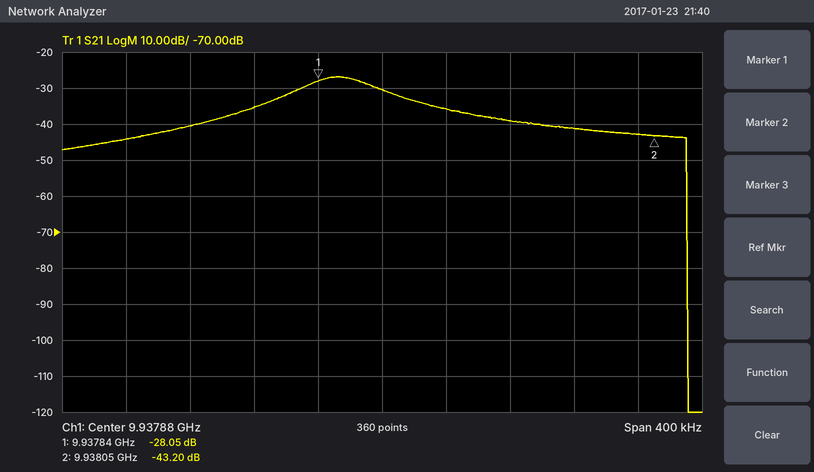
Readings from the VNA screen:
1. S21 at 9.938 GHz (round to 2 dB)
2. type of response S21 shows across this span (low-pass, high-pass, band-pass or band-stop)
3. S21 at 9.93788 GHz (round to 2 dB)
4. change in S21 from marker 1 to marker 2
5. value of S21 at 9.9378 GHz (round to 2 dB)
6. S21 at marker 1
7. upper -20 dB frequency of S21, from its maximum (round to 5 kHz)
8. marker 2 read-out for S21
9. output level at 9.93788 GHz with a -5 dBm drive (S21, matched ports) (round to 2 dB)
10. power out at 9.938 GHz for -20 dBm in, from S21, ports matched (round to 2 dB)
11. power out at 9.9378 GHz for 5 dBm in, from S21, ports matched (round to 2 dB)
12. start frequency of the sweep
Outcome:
-42 dB
band-pass
-30 dB
-15.15 dB
-36 dB
-28.05 dB
9.938070 GHz
-43.20 dB
-36 dBm
-62 dBm
-30 dBm
9.93768 GHz
